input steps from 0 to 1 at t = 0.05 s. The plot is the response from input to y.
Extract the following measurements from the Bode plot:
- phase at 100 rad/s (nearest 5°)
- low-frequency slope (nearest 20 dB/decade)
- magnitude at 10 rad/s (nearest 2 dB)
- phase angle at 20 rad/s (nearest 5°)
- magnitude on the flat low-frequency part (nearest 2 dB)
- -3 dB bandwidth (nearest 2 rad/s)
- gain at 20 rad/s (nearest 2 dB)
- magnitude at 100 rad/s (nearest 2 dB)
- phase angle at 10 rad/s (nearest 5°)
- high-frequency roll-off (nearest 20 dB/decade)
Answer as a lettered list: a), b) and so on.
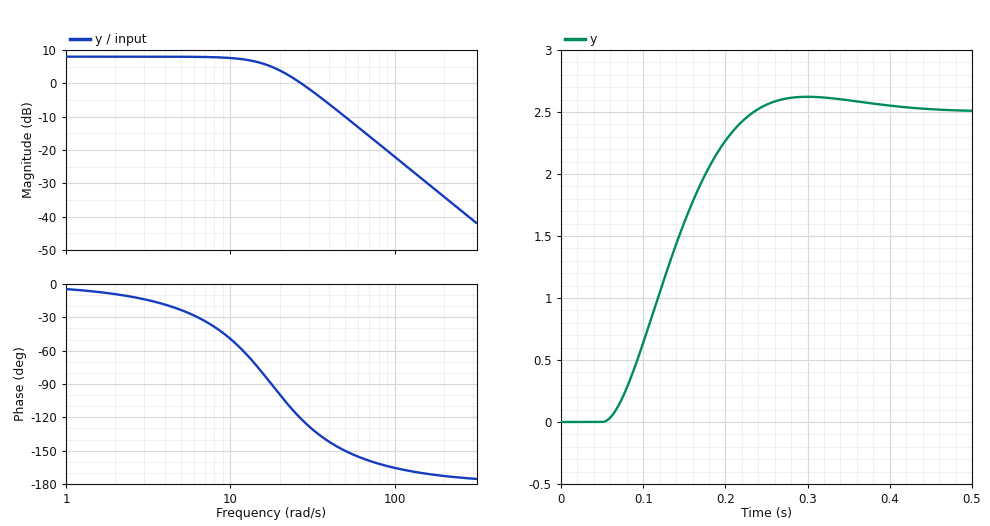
a) -165°
b) 0 dB/decade
c) 8 dB
d) -100°
e) 8 dB
f) 18 rad/s
g) 4 dB
h) -22 dB
i) -50°
j) -40 dB/decade
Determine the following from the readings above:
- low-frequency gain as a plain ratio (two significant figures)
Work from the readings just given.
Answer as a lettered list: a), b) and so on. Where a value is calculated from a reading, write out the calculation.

a) 10^(8 / 20) = 2.5
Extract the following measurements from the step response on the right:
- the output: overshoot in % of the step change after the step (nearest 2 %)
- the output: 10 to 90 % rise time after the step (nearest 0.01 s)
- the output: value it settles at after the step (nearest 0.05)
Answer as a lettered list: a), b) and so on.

a) 4 %
b) 0.12 s
c) 2.50
